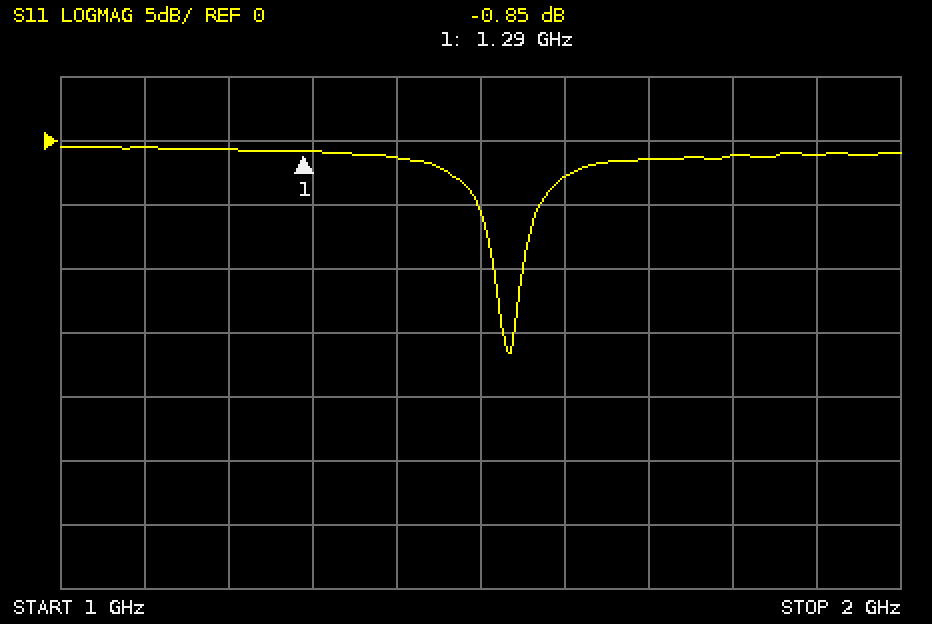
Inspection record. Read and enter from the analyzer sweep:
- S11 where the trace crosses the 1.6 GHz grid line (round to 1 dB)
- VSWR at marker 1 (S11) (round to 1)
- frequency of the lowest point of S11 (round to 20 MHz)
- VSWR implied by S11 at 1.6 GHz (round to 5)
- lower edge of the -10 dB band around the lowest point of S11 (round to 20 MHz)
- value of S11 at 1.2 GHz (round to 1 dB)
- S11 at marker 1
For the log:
-3 dB
20
1.54 GHz
5
1.52 GHz
-1 dB
-0.85 dB
